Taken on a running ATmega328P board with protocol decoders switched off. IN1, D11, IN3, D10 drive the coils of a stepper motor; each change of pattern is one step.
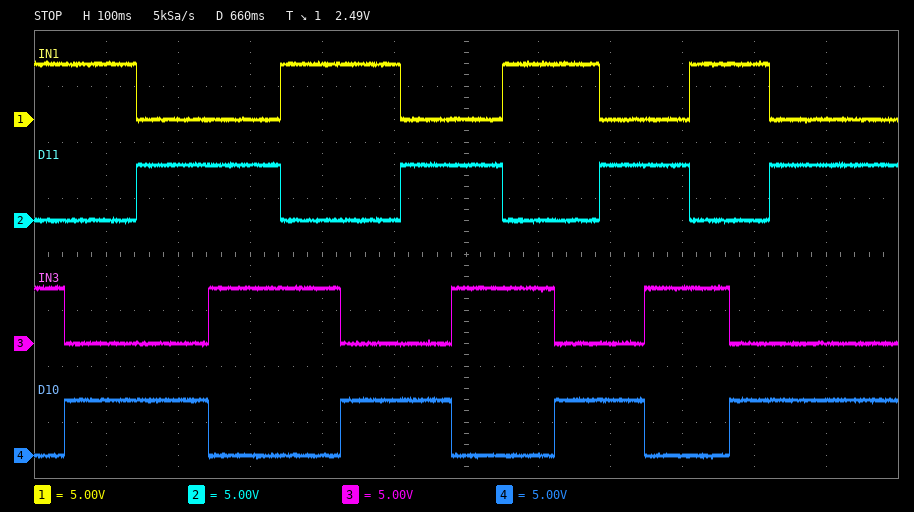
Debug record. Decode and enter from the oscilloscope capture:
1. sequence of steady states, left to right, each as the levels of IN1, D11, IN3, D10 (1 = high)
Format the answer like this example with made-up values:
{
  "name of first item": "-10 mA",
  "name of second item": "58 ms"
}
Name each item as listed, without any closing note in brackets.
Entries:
{
  "sequence of steady states, left to right, each as the levels of IN1, D11, IN3, D10": "1010 1001 0101 0110 1010 1001 0101 0110 1010 1001 0101 0110 1010 1001 0101"
}
